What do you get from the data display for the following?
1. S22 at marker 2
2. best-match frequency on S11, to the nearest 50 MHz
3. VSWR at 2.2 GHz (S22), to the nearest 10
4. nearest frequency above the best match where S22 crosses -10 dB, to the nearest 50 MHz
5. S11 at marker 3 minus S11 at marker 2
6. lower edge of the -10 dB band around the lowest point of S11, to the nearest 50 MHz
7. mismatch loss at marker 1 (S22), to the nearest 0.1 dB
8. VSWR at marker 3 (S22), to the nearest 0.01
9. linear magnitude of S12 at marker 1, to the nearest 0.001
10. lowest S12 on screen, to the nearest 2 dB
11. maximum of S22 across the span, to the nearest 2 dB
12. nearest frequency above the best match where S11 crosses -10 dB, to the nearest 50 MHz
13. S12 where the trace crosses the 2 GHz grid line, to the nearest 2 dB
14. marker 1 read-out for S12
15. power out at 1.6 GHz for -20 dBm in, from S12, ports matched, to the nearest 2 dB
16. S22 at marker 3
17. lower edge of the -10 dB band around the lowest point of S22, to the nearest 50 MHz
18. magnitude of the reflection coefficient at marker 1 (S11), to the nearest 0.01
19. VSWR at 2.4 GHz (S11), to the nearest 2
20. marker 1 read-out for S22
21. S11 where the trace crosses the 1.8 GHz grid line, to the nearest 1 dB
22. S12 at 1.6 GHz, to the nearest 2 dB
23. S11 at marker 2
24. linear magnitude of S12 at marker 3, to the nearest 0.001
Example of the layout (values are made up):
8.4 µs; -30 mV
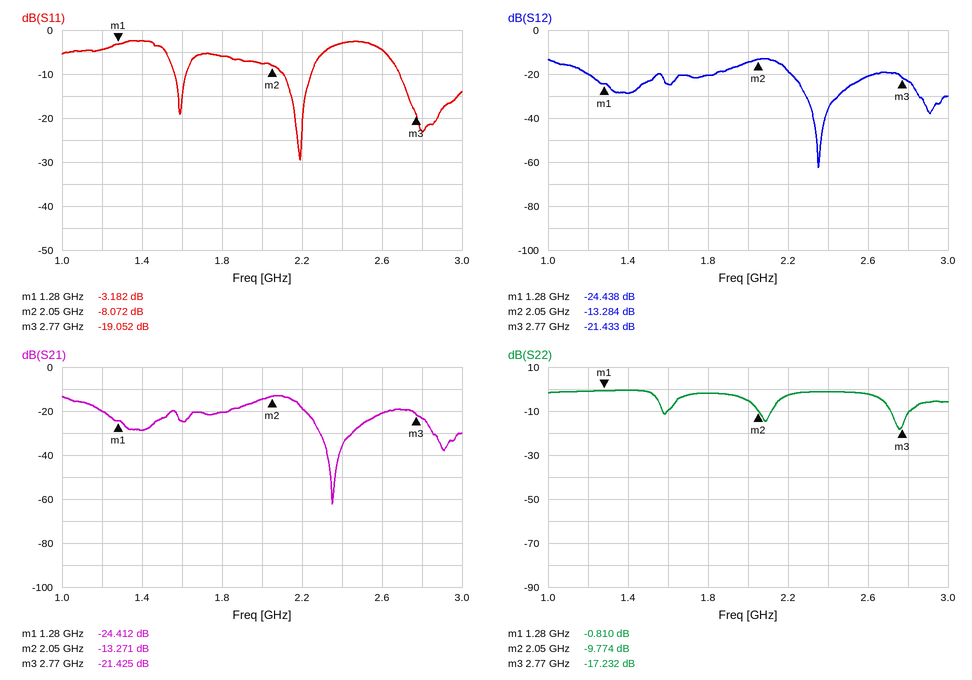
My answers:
-9.774 dB; 2.20 GHz; 10; 2.80 GHz; -10.980 dB; 2.10 GHz; 7.7 dB; 1.32; 0.060; -62 dB; 0 dB; 2.25 GHz; -14 dB; -24.438 dB; -44 dBm; -17.232 dB; 2.70 GHz; 0.69; 6; -0.810 dB; -6 dB; -24 dB; -8.072 dB; 0.085
